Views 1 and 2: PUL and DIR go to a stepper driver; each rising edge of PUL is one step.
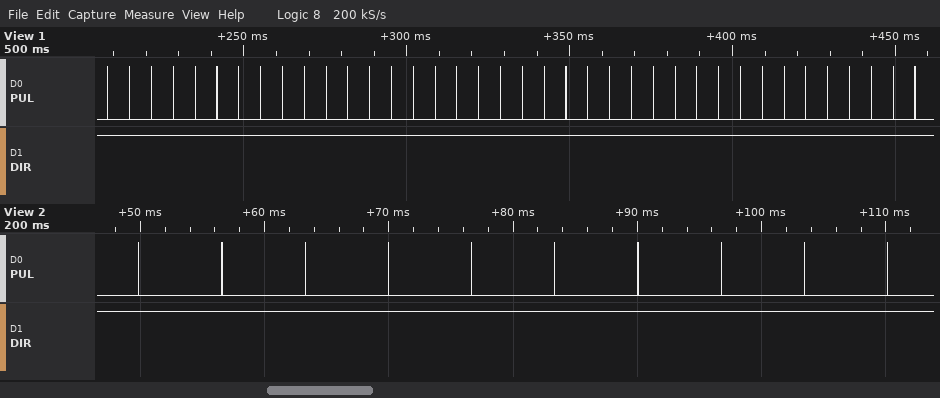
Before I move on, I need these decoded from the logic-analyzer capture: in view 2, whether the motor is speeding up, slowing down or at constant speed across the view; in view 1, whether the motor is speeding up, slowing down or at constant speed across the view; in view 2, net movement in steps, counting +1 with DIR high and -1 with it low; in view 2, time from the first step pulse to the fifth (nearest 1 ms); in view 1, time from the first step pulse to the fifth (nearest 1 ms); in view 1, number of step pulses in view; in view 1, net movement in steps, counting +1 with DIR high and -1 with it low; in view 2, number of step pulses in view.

constant speed
constant speed
+10
27 ms
27 ms
38
+38
10
